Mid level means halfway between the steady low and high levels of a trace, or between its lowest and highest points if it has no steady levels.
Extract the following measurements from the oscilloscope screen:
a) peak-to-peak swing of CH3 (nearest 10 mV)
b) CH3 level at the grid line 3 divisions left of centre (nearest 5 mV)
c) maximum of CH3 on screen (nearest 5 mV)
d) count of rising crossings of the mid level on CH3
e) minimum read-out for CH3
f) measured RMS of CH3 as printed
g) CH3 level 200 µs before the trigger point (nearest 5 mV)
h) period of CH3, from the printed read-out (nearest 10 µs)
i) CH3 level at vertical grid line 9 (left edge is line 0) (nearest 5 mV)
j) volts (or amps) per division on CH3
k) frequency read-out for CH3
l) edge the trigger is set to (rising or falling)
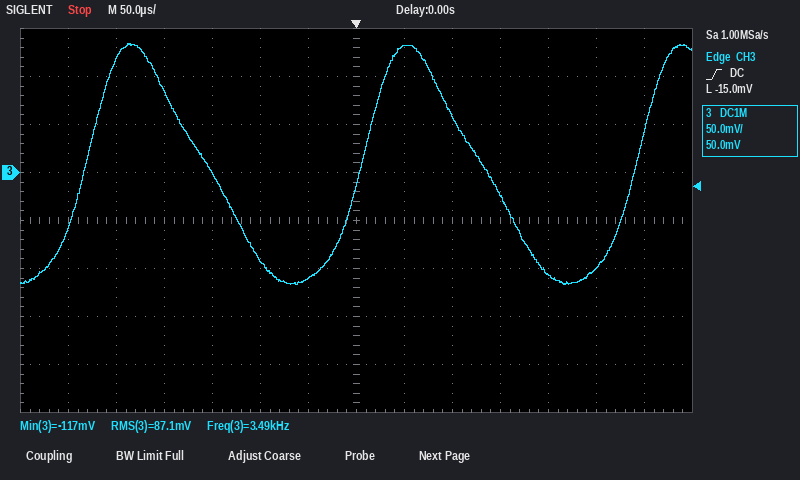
250 mV
0 mV
135 mV
3
-117 mV
87.1 mV
85 mV
290 µs
60 mV
50 mV
3.49 kHz
rising
